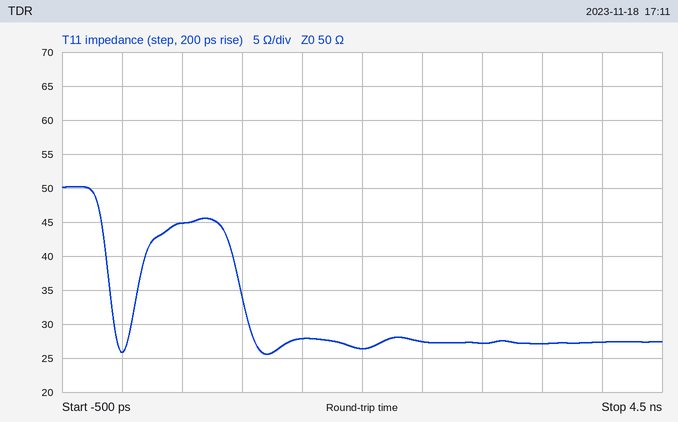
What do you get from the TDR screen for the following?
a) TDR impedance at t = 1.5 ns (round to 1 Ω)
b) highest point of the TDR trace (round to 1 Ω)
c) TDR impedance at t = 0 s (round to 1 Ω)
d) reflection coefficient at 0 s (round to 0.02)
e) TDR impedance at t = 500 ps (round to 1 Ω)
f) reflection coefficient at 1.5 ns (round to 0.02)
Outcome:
28 Ω
50 Ω
26 Ω
-0.32
45 Ω
-0.28
